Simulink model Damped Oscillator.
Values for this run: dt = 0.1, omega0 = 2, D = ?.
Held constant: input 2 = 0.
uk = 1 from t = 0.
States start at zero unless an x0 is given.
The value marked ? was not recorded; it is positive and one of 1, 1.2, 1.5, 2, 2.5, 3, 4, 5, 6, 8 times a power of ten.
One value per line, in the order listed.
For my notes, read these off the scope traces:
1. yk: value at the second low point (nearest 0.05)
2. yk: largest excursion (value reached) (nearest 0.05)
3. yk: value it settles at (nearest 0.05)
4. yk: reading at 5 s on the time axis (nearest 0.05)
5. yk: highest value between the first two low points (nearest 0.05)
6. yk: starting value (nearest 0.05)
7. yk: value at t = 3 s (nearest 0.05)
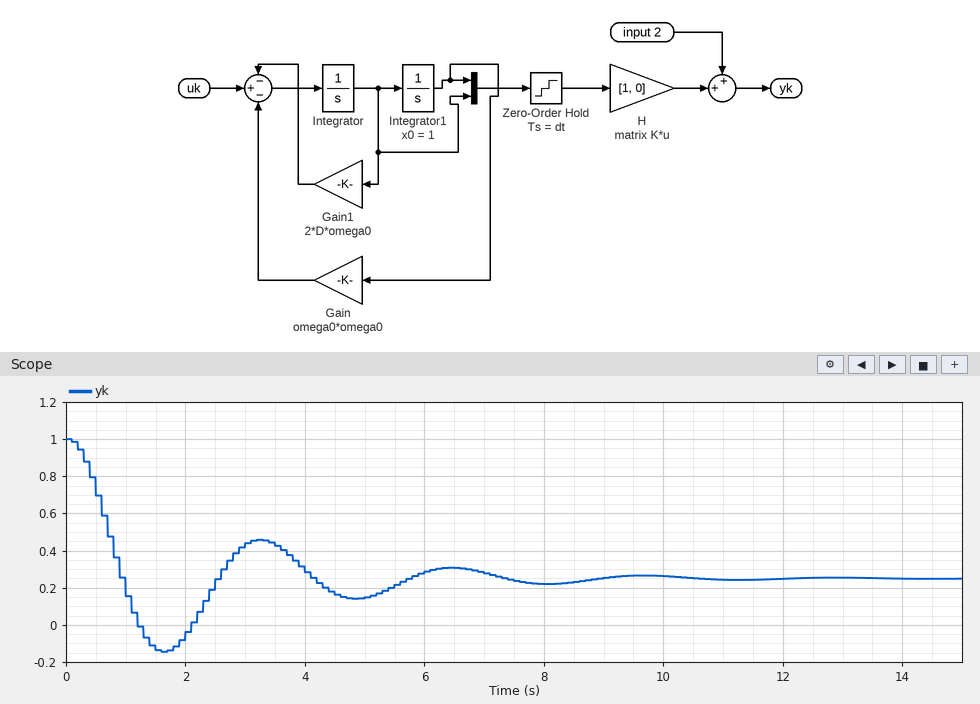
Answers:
0.15
-0.15
0.25
0.15
0.45
1.00
0.45
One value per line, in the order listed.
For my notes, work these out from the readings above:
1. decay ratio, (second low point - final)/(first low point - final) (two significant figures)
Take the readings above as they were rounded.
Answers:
0.25
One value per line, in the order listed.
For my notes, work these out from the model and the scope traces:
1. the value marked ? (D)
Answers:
0.2
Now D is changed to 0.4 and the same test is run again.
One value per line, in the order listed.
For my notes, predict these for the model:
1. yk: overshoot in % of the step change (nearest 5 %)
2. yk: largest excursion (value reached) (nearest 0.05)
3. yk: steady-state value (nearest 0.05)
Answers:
25 %
0.05
0.25
